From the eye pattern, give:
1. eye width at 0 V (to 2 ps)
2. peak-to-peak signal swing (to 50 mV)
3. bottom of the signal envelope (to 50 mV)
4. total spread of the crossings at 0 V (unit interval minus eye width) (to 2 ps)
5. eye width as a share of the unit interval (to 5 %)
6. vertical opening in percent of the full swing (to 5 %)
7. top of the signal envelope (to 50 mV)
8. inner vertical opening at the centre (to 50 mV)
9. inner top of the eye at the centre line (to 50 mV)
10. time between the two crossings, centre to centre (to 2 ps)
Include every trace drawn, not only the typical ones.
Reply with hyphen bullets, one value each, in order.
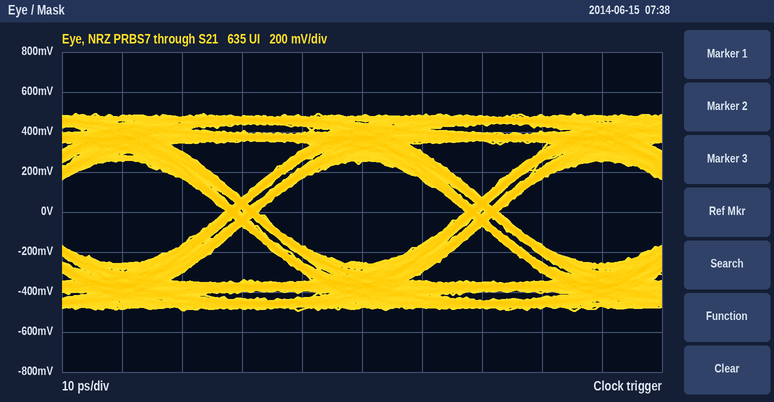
- 34 ps
- 1.00 V
- -500 mV
- 6 ps
- 85 %
- 50 %
- 500 mV
- 500 mV
- 250 mV
- 40 ps
